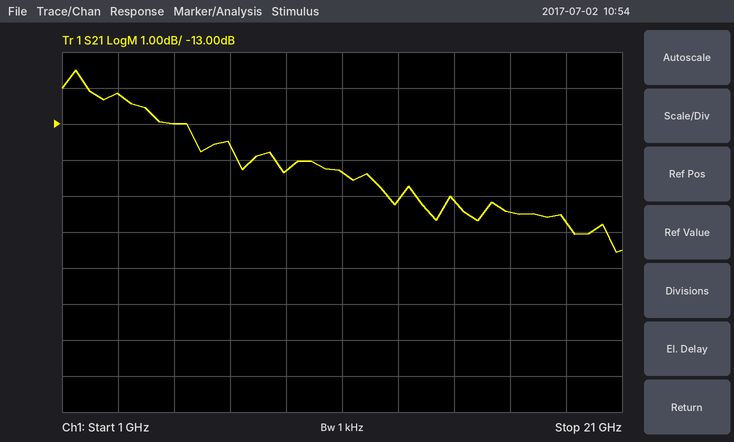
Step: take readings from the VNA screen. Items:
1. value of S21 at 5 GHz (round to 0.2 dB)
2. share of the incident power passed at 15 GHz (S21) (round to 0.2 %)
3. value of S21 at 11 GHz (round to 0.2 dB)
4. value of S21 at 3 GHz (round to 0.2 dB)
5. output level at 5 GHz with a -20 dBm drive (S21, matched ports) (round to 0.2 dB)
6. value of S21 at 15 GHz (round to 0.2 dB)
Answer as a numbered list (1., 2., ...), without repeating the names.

1. -13.0 dB
2. 3.0 %
3. -14.4 dB
4. -12.2 dB
5. -33.0 dBm
6. -15.2 dB
